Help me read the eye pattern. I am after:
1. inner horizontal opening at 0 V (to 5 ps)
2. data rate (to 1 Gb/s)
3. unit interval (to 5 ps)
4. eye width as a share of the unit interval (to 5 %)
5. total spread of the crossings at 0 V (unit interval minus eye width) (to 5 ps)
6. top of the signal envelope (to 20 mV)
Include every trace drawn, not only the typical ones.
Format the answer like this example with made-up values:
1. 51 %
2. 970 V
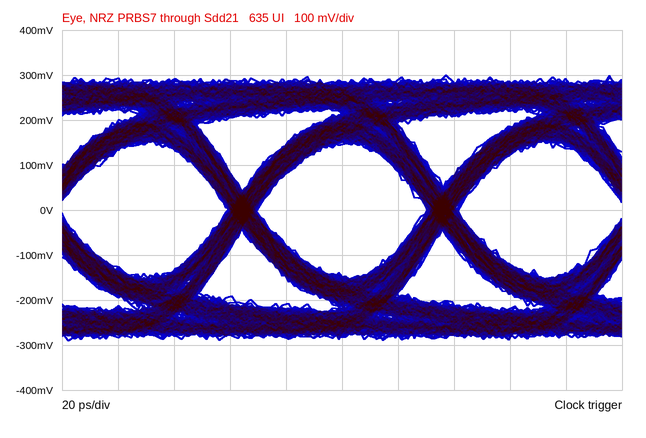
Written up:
1. 60 ps
2. 14 Gb/s
3. 70 ps
4. 85 %
5. 10 ps
6. 300 mV
